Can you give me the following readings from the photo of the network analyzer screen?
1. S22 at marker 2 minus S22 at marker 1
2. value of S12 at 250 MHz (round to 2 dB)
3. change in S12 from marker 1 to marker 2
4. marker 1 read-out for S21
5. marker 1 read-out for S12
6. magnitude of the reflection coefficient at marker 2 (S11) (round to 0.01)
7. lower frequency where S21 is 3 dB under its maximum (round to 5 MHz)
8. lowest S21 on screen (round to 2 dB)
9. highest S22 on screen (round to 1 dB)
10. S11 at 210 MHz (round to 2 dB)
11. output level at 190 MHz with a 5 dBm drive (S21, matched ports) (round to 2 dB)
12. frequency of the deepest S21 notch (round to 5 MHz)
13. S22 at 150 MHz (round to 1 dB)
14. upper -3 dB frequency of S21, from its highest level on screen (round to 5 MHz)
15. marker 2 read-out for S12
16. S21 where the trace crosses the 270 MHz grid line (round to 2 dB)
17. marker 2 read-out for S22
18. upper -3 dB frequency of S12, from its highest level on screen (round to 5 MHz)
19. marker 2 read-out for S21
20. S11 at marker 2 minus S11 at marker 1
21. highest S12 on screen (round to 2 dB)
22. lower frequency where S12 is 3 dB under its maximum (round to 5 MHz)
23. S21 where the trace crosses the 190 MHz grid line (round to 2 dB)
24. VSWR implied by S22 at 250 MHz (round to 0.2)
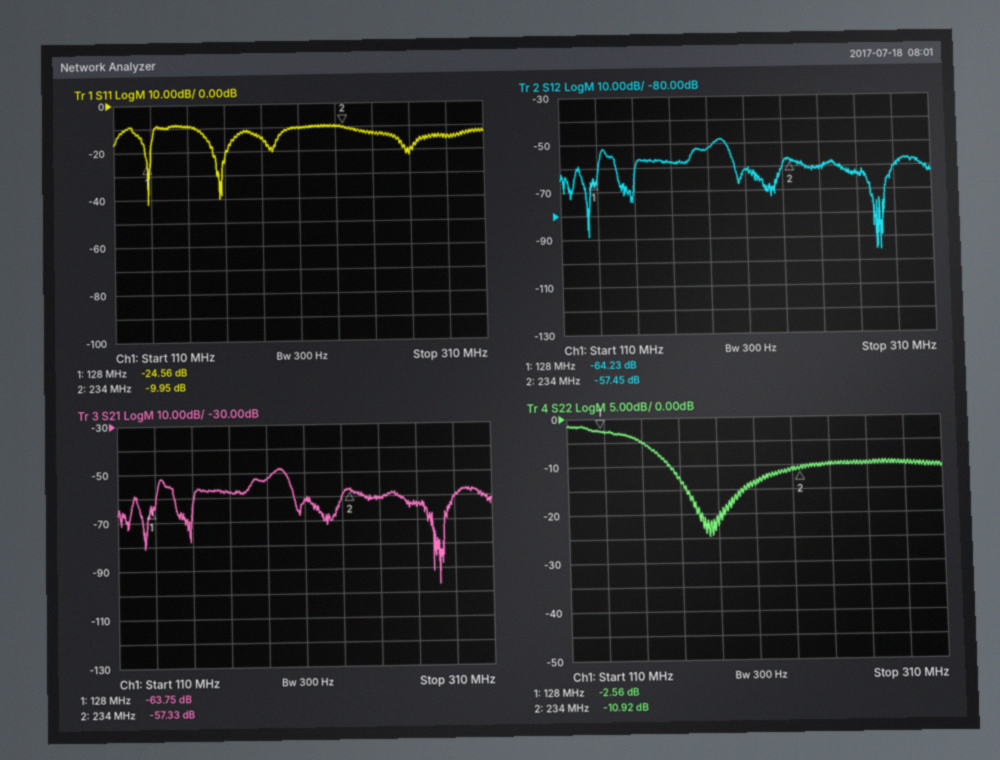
-8.36 dB
-60 dB
6.78 dB
-63.75 dB
-64.23 dB
0.32
190 MHz
-96 dB
-1 dB
-10 dB
-48 dBm
280 MHz
-5 dB
200 MHz
-57.45 dB
-64 dB
-10.92 dB
200 MHz
-57.33 dB
14.61 dB
-48 dB
190 MHz
-52 dB
2.0
